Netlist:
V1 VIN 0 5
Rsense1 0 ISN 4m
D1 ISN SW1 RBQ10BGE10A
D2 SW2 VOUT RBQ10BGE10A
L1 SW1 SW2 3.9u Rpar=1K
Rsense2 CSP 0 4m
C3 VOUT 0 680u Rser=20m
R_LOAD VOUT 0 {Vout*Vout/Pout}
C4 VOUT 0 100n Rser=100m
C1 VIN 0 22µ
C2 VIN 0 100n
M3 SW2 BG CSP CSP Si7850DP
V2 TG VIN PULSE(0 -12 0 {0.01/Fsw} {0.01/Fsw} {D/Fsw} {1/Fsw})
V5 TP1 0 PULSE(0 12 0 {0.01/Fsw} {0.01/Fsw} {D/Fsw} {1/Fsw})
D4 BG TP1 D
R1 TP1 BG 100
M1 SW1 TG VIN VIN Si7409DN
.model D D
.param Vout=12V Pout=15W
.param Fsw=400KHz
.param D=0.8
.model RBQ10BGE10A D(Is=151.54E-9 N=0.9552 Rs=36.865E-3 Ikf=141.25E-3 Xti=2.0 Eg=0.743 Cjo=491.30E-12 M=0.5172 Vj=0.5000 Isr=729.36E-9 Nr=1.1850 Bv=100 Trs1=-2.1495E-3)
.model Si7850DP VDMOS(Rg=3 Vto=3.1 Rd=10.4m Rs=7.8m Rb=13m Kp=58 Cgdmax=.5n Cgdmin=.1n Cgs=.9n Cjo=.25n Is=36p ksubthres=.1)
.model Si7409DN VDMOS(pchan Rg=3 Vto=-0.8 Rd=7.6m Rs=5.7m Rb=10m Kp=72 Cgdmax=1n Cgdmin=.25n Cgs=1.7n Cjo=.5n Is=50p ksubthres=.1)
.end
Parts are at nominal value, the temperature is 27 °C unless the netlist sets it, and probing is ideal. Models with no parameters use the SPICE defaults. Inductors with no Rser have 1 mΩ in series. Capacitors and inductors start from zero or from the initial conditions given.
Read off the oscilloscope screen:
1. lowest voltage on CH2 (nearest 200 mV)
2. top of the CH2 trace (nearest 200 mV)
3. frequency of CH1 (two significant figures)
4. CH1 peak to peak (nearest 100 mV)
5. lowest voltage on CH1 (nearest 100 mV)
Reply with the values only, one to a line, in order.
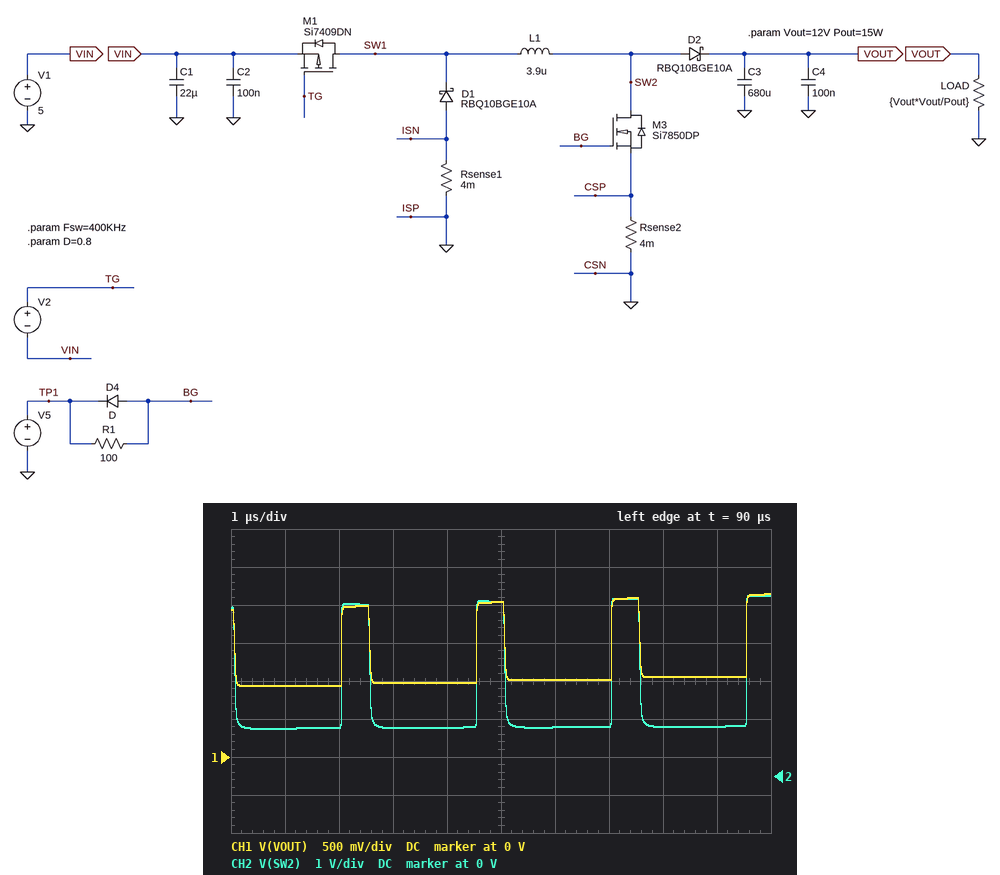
1.2 V
4.8 V
400 kHz
1.2 V
900 mV
